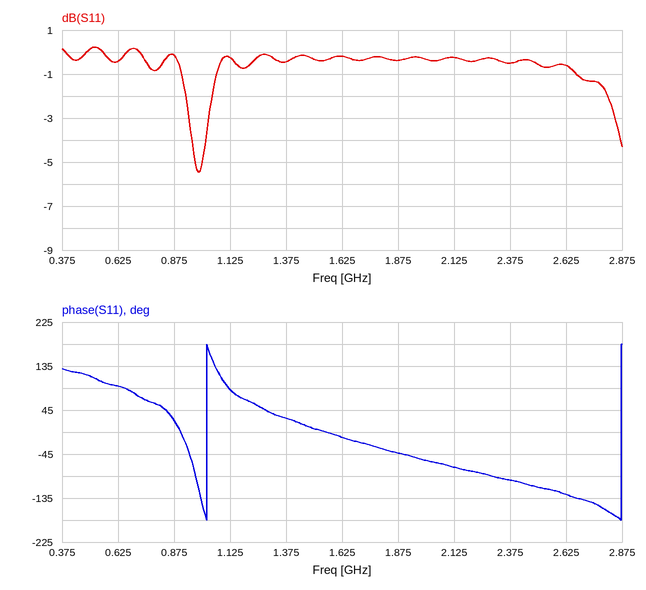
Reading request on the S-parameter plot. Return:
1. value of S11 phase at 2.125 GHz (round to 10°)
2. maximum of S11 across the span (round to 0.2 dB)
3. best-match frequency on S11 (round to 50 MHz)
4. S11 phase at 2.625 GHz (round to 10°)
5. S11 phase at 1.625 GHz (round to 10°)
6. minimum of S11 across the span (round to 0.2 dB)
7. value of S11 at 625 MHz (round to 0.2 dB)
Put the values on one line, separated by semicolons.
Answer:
-70°; 0.2 dB; 1.00 GHz; -130°; -10°; -5.4 dB; -0.4 dB
